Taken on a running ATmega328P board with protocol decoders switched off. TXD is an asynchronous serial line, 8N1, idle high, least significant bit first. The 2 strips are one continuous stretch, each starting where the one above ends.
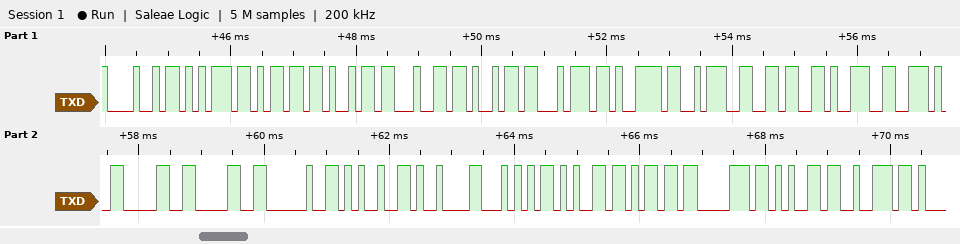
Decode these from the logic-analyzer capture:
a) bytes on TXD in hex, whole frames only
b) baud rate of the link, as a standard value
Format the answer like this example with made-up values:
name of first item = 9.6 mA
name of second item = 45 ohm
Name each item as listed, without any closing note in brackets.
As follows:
bytes on TXD in hex, whole frames only = 48 75 6D 69 64 69 74 79 3A 36 39 2E 30 30 20 25 09 54 65 6D 70 65 72
baud rate of the link, as a standard value = 9600 baud
